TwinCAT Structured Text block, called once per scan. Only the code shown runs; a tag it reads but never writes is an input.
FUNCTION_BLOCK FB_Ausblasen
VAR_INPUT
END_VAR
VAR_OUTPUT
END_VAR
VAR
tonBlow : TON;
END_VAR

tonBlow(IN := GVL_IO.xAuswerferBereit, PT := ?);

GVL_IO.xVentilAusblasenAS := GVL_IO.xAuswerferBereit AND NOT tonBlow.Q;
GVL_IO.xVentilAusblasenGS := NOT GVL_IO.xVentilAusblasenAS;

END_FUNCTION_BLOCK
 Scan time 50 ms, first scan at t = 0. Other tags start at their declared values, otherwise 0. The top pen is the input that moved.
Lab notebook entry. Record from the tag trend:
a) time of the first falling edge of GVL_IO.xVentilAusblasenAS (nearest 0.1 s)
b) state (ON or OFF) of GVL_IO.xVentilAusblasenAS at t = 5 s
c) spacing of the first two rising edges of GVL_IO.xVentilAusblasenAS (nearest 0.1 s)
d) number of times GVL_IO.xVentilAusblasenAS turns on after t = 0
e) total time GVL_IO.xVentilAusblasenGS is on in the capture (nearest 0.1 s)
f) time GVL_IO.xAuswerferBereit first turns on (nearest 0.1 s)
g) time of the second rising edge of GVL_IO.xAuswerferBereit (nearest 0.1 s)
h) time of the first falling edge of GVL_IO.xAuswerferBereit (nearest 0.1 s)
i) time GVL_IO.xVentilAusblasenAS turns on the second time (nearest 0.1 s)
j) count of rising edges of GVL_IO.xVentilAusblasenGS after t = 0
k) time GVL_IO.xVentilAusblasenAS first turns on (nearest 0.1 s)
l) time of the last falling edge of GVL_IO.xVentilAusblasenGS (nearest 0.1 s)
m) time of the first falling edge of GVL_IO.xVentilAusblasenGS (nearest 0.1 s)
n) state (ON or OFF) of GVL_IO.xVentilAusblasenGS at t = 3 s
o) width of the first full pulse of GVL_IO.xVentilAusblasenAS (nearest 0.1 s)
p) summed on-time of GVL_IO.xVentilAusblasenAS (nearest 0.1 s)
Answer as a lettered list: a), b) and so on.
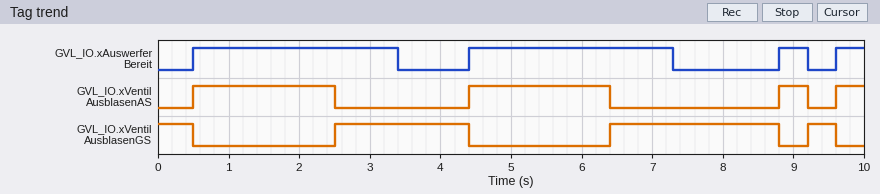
a) 2.5 s
b) ON
c) 3.9 s
d) 4
e) 5.2 s
f) 0.5 s
g) 4.4 s
h) 3.4 s
i) 4.4 s
j) 3
k) 0.5 s
l) 9.6 s
m) 0.5 s
n) ON
o) 2.0 s
p) 4.8 s
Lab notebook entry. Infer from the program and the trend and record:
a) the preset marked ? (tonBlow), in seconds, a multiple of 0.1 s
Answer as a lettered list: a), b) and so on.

a) 2.0 s
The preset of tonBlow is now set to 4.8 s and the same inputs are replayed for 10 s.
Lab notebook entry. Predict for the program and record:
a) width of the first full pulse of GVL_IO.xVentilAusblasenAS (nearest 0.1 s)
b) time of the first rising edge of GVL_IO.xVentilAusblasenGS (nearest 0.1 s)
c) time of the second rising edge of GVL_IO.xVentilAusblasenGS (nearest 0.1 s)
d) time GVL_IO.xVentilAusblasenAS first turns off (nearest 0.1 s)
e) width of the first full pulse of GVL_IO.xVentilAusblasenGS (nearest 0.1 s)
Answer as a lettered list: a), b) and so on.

a) 2.9 s
b) 3.4 s
c) 7.3 s
d) 3.4 s
e) 1.0 s
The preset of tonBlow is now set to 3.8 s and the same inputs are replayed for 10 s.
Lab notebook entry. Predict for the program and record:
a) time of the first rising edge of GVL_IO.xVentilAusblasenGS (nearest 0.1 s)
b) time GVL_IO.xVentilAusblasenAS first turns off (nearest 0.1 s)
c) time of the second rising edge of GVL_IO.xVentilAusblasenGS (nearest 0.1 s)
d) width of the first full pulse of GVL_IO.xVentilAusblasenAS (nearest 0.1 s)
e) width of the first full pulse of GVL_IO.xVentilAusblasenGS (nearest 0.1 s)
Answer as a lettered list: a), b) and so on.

a) 3.4 s
b) 3.4 s
c) 7.3 s
d) 2.9 s
e) 1.0 s
